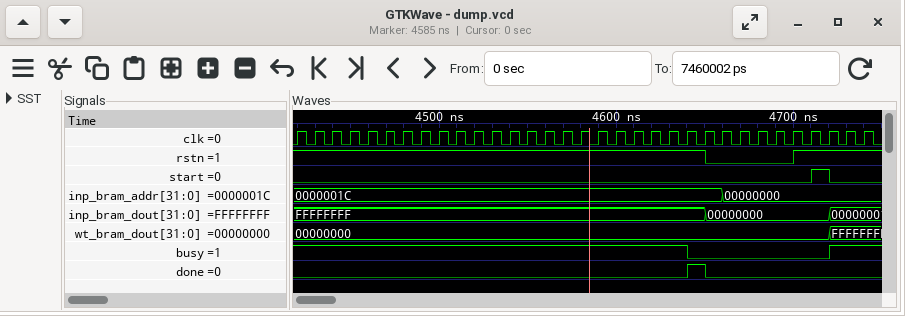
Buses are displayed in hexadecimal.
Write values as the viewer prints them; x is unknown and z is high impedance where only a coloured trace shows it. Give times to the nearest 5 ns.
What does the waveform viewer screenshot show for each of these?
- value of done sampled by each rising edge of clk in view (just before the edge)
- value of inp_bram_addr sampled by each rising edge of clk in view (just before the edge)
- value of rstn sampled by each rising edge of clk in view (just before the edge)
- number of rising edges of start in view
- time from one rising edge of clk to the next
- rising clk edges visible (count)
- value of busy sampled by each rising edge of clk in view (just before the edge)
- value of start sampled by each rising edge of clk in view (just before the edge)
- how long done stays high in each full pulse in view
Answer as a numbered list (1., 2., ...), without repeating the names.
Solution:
1. 0 0 0 0 0 0 0 0 0 0 0 0 0 0 0 0 0 0 0 0 0 0 0 1 0 0 0 0 0 0 0 0 0
2. 0000001C, 0000001C, 0000001C, 0000001C, 0000001C, 0000001C, 0000001C, 0000001C, 0000001C, 0000001C, 0000001C, 0000001C, 0000001C, 0000001C, 0000001C, 0000001C, 0000001C, 0000001C, 0000001C, 0000001C, 0000001C, 0000001C, 0000001C, 0000001C, 0000001C, 00000000, 00000000, 00000000, 00000000, 00000000, 00000000, 00000000, 00000000
3. 1 1 1 1 1 1 1 1 1 1 1 1 1 1 1 1 1 1 1 1 1 1 1 1 0 0 0 0 0 1 1 1 1
4. 1
5. 10 ns
6. 33
7. 1 1 1 1 1 1 1 1 1 1 1 1 1 1 1 1 1 1 1 1 1 1 1 0 0 0 0 0 0 0 0 1 1
8. 0 0 0 0 0 0 0 0 0 0 0 0 0 0 0 0 0 0 0 0 0 0 0 0 0 0 0 0 0 0 1 0 0
9. 10 ns
